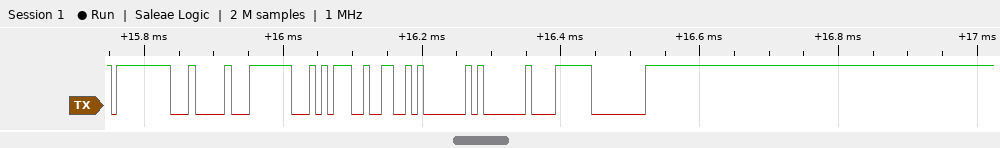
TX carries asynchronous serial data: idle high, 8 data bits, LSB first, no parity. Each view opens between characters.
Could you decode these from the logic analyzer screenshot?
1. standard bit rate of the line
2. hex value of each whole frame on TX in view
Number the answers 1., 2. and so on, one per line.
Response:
1. 115200 baud
2. FF, 04, FC, D4, 32, 01, 01, F8, 00
